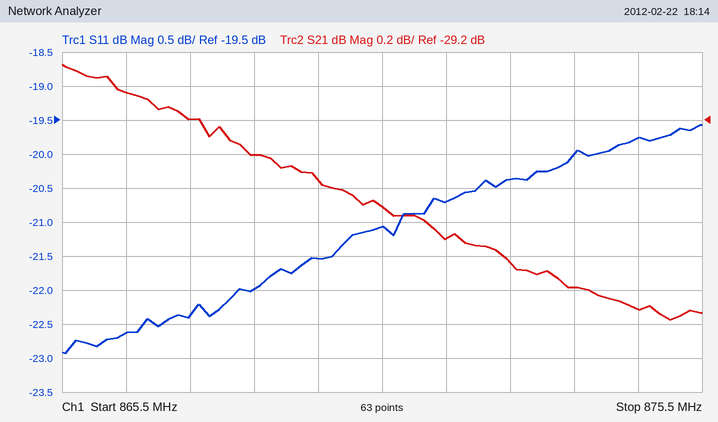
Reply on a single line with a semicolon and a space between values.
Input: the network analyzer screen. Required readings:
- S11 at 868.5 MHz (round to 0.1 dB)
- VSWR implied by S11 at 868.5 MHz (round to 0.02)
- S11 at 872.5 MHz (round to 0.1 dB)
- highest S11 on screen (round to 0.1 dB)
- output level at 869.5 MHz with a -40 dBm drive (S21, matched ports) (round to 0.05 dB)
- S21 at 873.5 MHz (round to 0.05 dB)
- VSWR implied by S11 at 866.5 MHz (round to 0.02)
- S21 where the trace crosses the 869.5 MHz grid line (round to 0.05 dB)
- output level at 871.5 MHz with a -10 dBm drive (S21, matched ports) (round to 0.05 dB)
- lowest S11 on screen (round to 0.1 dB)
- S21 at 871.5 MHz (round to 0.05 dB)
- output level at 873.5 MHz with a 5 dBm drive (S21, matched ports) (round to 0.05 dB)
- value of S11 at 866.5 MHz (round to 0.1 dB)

-22.0 dB; 1.18; -20.4 dB; -19.6 dB; -69.55 dBm; -30.20 dB; 1.16; -29.55 dB; -39.90 dBm; -22.9 dB; -29.90 dB; -25.20 dBm; -22.6 dB
